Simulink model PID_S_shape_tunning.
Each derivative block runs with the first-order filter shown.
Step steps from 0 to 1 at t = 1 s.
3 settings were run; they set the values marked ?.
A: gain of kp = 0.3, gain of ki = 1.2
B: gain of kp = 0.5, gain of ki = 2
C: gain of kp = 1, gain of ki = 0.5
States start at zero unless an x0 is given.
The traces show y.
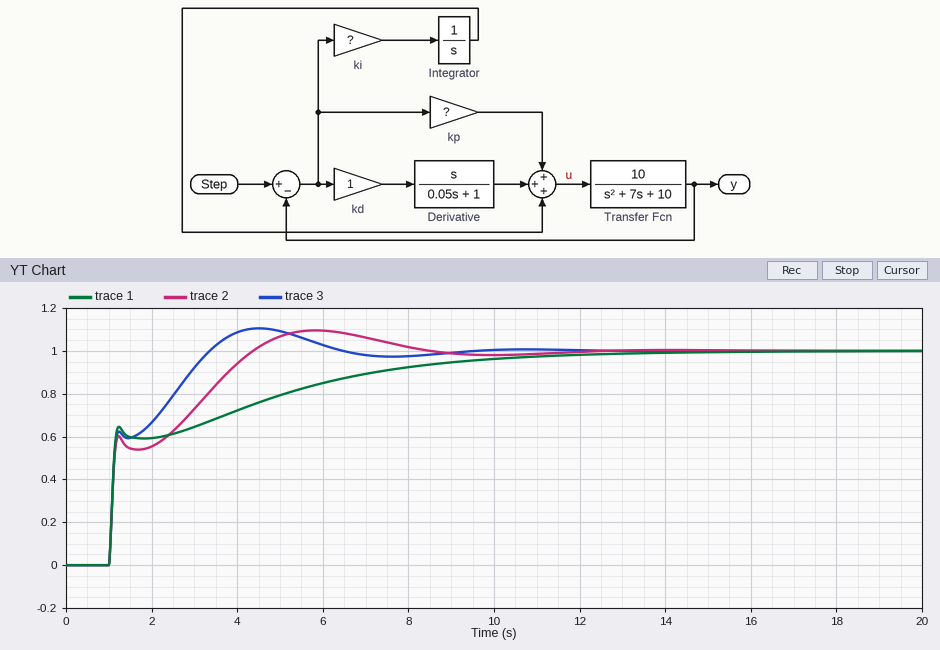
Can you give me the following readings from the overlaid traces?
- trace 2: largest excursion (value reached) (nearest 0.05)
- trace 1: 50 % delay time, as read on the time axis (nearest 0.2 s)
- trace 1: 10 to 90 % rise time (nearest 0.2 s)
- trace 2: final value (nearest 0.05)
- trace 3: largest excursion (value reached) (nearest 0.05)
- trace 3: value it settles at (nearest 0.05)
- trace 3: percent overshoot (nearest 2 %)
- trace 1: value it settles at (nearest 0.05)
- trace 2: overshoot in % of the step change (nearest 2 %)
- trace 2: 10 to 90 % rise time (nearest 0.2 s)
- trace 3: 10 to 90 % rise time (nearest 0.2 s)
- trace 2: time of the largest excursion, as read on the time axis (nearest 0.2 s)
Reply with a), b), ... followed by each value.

a) 1.10
b) 1.2 s
c) 6.2 s
d) 1.00
e) 1.10
f) 1.00
g) 10 %
h) 1.00
i) 10 %
j) 2.8 s
k) 1.8 s
l) 5.8 s
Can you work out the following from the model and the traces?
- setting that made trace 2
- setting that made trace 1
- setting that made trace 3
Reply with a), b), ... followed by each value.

a) A
b) C
c) B
